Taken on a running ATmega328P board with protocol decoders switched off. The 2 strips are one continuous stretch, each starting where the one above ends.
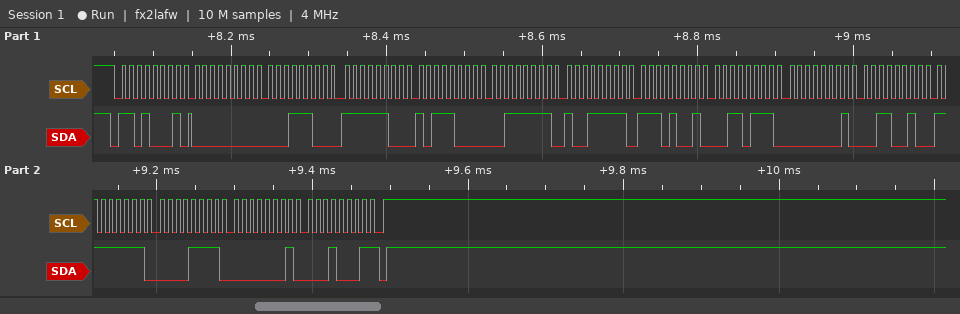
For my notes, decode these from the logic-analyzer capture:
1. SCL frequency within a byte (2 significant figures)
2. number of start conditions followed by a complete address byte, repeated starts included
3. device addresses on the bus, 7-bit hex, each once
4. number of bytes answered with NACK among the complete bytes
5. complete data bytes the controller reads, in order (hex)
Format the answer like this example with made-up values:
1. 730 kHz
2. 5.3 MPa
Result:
1. 100 kHz
2. 1
3. 0x68
4. 1
5. 00 1C FC B8 3F 9F E9 37 01 32 FF 0F 01 11
